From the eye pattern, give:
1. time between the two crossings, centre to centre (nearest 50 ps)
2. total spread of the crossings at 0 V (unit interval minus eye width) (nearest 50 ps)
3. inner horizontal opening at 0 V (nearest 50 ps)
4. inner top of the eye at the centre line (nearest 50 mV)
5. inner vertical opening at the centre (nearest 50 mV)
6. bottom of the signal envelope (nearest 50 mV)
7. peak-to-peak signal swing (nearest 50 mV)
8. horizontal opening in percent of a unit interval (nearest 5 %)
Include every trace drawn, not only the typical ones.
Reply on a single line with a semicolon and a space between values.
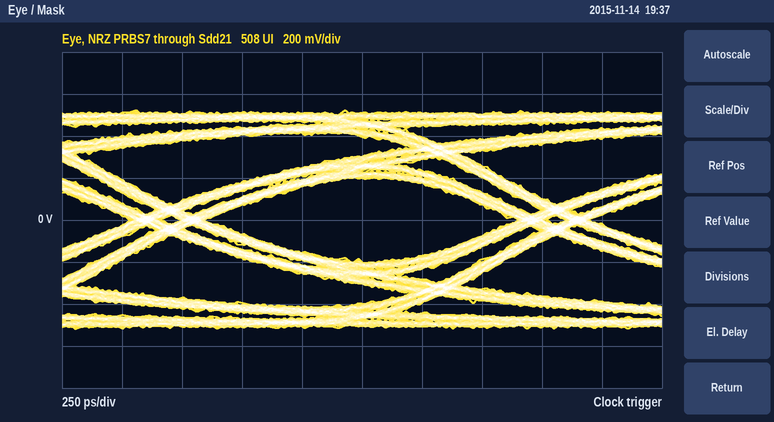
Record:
1.60 ns; 300 ps; 1.30 ns; 200 mV; 400 mV; -500 mV; 1.05 V; 80 %
